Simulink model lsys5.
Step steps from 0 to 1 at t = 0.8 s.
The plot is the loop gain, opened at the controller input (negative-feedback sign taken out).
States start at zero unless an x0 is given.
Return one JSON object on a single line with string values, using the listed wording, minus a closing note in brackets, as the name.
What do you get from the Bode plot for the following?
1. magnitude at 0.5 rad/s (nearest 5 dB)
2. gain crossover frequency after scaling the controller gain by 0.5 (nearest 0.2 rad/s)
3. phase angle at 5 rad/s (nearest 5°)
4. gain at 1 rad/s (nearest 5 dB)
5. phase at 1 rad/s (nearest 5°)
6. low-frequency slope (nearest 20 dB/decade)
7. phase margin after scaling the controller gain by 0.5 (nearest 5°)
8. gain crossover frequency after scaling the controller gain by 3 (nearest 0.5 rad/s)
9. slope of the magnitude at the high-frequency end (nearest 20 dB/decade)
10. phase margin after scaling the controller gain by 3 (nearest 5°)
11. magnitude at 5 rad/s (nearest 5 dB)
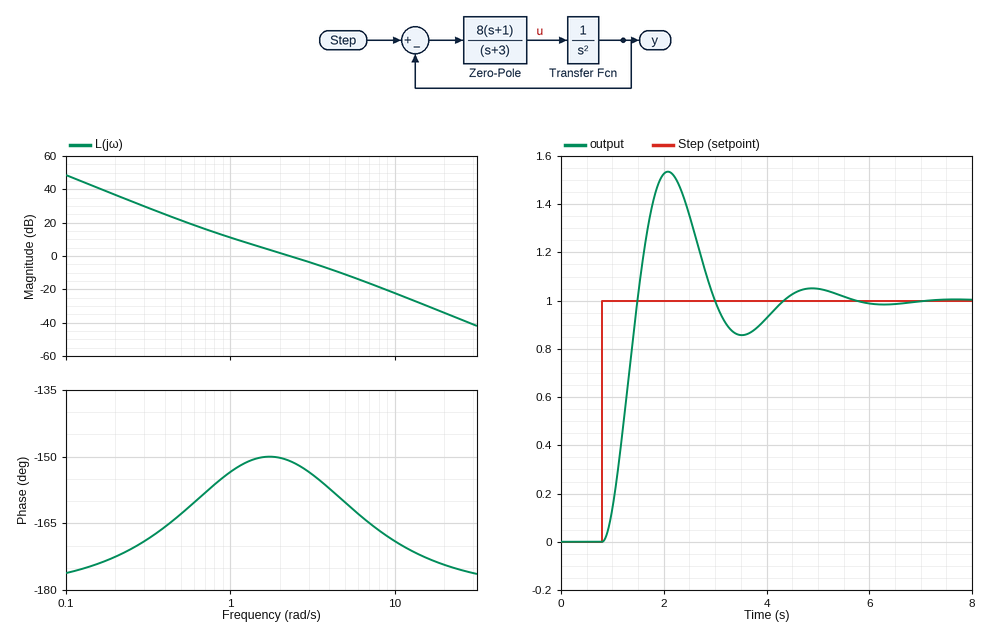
{"magnitude at 0.5 rad/s": "20 dB", "gain crossover frequency after scaling the controller gain by 0.5": "1.4 rad/s", "phase angle at 5 rad/s": "-160°", "gain at 1 rad/s": "10 dB", "phase at 1 rad/s": "-155°", "low-frequency slope": "-40 dB/decade", "phase margin after scaling the controller gain by 0.5": "30°", "gain crossover frequency after scaling the controller gain by 3": "4.5 rad/s", "slope of the magnitude at the high-frequency end": "-40 dB/decade", "phase margin after scaling the controller gain by 3": "20°", "magnitude at 5 rad/s": "-10 dB"}
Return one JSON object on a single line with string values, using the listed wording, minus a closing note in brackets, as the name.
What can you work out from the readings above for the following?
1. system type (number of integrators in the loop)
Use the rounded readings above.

{"system type": "2"}
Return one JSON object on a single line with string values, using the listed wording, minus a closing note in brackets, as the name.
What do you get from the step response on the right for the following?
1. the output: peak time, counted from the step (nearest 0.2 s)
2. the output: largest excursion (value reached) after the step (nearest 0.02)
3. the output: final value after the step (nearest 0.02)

{"the output: peak time, counted from the step": "1.2 s", "the output: largest excursion (value reached) after the step": "1.54", "the output: final value after the step": "1.00"}
